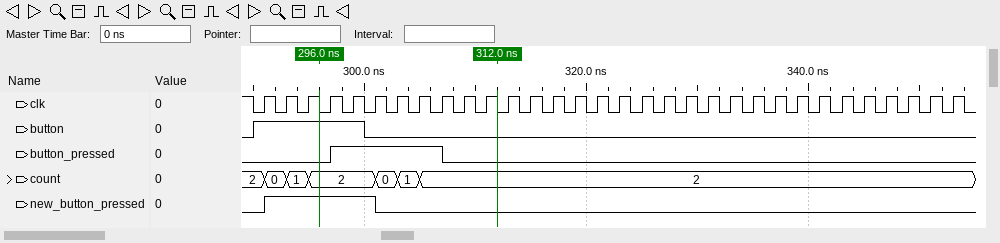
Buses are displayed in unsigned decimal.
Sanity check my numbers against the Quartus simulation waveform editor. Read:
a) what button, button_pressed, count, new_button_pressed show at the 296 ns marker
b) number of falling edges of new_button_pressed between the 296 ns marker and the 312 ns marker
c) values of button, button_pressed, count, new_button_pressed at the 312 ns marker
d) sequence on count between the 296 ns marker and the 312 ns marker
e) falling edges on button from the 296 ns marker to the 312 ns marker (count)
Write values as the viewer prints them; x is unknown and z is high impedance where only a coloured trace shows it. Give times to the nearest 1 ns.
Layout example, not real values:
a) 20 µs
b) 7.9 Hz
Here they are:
a) button=1, button_pressed=0, count=2, new_button_pressed=1
b) 1
c) button=0, button_pressed=0, count=2, new_button_pressed=0
d) 2, 0, 1, 2
e) 1
